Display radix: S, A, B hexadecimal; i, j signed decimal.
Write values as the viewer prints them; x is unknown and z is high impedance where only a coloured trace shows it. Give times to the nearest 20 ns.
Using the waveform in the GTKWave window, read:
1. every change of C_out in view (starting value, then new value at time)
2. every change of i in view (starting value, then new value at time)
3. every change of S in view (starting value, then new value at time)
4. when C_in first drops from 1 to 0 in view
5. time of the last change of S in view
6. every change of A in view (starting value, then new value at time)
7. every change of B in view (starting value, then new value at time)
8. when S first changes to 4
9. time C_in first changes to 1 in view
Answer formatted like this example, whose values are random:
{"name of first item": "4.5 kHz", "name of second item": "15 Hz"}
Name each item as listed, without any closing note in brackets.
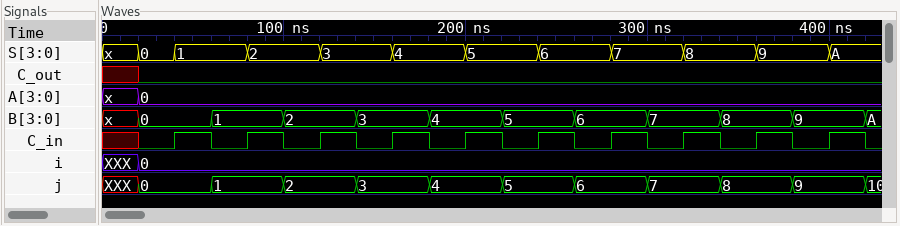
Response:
{"every change of C_out in view": "x, 0 at 20 ns", "every change of i in view": "XXX, 0 at 20 ns", "every change of S in view": "x, 0 at 20 ns, 1 at 40 ns, 2 at 80 ns, 3 at 120 ns, 4 at 160 ns, 5 at 200 ns, 6 at 240 ns, 7 at 280 ns, 8 at 320 ns, 9 at 360 ns, A at 400 ns", "when C_in first drops from 1 to 0 in view": "60 ns", "time of the last change of S in view": "400 ns", "every change of A in view": "x, 0 at 20 ns", "every change of B in view": "x, 0 at 20 ns, 1 at 60 ns, 2 at 100 ns, 3 at 140 ns, 4 at 180 ns, 5 at 220 ns, 6 at 260 ns, 7 at 300 ns, 8 at 340 ns, 9 at 380 ns, A at 420 ns", "when S first changes to 4": "160 ns", "time C_in first changes to 1 in view": "40 ns"}
